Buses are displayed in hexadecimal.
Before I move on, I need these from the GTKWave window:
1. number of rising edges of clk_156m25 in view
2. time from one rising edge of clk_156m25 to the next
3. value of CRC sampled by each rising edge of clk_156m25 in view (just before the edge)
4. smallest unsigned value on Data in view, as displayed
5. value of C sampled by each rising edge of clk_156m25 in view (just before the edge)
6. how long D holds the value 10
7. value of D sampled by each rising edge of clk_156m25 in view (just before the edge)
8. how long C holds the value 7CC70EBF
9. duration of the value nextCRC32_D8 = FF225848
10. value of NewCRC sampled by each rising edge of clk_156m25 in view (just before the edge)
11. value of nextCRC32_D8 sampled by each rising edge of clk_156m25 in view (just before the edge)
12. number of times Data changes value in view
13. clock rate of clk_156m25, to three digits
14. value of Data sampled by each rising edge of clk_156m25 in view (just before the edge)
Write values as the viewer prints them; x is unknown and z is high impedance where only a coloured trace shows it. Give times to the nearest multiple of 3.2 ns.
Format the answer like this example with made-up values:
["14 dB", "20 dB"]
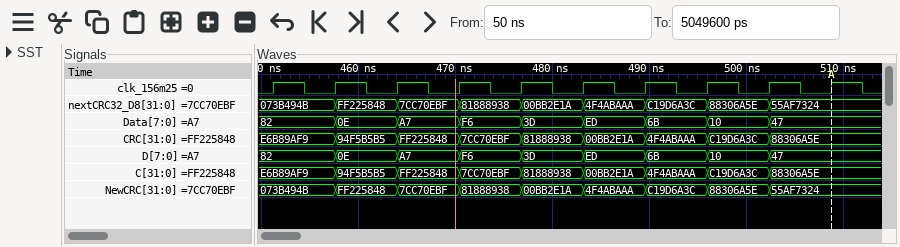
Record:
["10", "6.4 ns", "E6B89AF9, E6B89AF9, 94F5B5B5, FF225848, 7CC70EBF, 81888938, 00BB2E1A, 4F4ABAAA, C19D6A3C, 88306A5E", "0E", "E6B89AF9, E6B89AF9, 94F5B5B5, FF225848, 7CC70EBF, 81888938, 00BB2E1A, 4F4ABAAA, C19D6A3C, 88306A5E", "6.4 ns", "82, 82, 0E, A7, F6, 3D, ED, 6B, 10, 47", "6.4 ns", "6.4 ns", "073B494B, 073B494B, FF225848, 7CC70EBF, 81888938, 00BB2E1A, 4F4ABAAA, C19D6A3C, 88306A5E, 55AF7324", "073B494B, 073B494B, FF225848, 7CC70EBF, 81888938, 00BB2E1A, 4F4ABAAA, C19D6A3C, 88306A5E, 55AF7324", "8", "156 MHz", "82, 82, 0E, A7, F6, 3D, ED, 6B, 10, 47"]
